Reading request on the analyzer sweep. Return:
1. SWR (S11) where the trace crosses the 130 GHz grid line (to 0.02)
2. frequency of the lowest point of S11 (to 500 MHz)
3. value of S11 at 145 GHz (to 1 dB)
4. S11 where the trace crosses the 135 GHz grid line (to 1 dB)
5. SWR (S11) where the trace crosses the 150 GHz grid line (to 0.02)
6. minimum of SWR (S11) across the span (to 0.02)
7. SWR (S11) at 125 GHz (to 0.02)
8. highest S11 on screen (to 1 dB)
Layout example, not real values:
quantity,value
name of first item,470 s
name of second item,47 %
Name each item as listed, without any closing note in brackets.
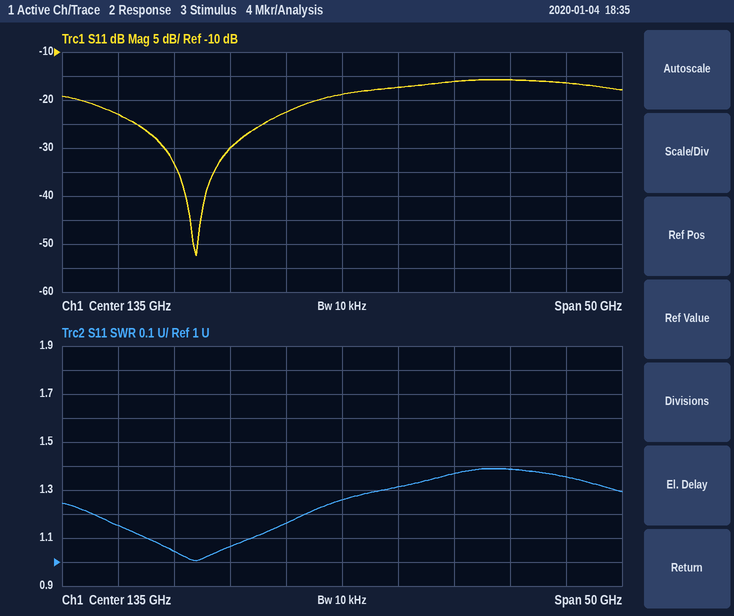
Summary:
quantity,value
SWR (S11) where the trace crosses the 130 GHz grid line,1.16
frequency of the lowest point of S11,122.0 GHz
value of S11 at 145 GHz,-16 dB
S11 where the trace crosses the 135 GHz grid line,-19 dB
SWR (S11) where the trace crosses the 150 GHz grid line,1.38
minimum of SWR (S11) across the span,1.00
SWR (S11) at 125 GHz,1.06
highest S11 on screen,-16 dB
